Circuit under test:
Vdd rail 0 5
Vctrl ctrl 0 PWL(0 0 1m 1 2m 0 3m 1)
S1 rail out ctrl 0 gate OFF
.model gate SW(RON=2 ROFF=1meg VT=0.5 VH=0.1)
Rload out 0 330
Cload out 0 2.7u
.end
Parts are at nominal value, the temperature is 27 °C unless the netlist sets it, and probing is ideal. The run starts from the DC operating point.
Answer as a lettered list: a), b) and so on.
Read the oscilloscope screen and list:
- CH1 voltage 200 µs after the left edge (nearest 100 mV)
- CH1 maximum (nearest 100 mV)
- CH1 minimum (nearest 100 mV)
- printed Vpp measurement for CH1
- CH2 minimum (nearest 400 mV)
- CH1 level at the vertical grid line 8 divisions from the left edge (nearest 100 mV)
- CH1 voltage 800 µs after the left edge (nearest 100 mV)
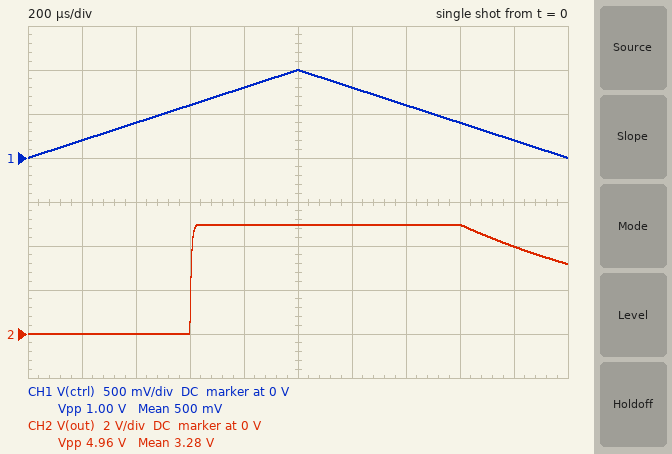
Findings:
a) 200 mV
b) 1.0 V
c) 0 V
d) 1.00 V
e) 0 V
f) 400 mV
g) 800 mV
